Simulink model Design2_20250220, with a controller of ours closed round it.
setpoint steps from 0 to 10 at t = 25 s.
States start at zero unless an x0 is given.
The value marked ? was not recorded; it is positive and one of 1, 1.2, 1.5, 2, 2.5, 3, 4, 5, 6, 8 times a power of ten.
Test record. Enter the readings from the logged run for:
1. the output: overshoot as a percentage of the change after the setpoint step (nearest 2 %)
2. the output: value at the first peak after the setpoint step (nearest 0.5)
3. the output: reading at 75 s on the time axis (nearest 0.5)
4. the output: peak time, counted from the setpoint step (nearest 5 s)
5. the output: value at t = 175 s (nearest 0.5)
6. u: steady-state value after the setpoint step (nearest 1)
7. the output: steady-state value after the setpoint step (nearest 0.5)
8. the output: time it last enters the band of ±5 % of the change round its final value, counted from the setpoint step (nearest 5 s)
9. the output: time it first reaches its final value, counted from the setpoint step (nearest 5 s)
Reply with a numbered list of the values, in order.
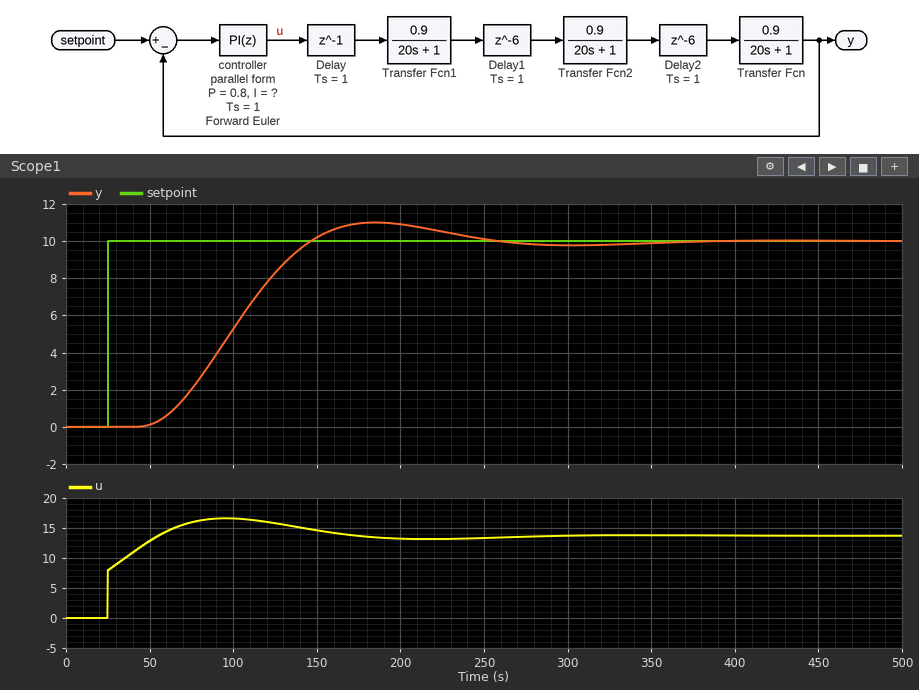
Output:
1. 10 %
2. 11.0
3. 2.0
4. 160 s
5. 11.0
6. 14
7. 10.0
8. 200 s
9. 120 s
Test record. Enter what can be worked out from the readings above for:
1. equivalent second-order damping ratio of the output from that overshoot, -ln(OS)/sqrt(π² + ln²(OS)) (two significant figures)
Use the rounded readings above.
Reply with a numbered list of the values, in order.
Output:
1. 0.59
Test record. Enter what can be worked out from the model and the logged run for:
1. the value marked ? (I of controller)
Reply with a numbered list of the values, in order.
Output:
1. 0.02
